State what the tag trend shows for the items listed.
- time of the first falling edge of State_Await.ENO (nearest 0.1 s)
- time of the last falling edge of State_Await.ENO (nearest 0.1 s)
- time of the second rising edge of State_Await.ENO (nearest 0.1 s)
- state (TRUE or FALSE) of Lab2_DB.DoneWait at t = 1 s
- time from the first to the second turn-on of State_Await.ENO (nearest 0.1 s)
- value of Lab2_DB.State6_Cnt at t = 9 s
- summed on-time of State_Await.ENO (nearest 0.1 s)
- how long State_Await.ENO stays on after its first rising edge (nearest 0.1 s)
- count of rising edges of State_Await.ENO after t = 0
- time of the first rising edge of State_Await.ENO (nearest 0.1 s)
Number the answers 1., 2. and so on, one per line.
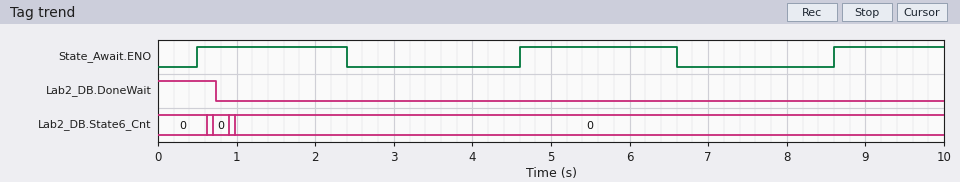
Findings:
1. 2.4 s
2. 6.6 s
3. 4.6 s
4. FALSE
5. 4.1 s
6. 0
7. 5.3 s
8. 1.9 s
9. 3
10. 0.5 s
